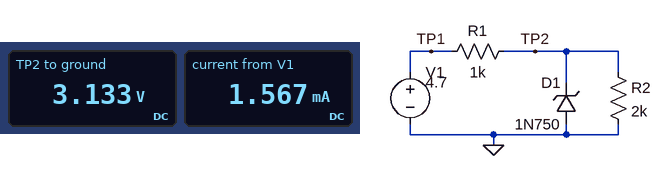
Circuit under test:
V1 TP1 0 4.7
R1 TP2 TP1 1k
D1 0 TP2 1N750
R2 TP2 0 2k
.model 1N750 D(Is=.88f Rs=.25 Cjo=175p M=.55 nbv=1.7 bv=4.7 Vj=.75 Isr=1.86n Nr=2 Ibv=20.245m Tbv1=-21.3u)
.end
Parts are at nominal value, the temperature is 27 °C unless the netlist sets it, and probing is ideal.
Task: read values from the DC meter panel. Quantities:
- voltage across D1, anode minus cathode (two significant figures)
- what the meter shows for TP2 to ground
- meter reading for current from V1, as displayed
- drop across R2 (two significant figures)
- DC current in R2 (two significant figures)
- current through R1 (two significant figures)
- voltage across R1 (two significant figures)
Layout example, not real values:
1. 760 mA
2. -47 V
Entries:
1. -3.1 V
2. 3.133 V
3. 1.567 mA
4. 3.1 V
5. 1.6 mA
6. 1.6 mA
7. 1.6 V
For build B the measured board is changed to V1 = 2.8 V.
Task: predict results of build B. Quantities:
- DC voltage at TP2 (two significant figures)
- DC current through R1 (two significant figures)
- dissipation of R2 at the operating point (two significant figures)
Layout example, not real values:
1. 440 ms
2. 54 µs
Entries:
1. 1.9 V
2. 930 µA
3. 1.7 mW
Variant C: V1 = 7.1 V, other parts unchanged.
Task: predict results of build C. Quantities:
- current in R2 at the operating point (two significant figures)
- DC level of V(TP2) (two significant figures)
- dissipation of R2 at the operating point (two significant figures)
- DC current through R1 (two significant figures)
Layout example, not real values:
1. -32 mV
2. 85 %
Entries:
1. 2.3 mA
2. 4.5 V
3. 10 mW
4. 2.6 mA
